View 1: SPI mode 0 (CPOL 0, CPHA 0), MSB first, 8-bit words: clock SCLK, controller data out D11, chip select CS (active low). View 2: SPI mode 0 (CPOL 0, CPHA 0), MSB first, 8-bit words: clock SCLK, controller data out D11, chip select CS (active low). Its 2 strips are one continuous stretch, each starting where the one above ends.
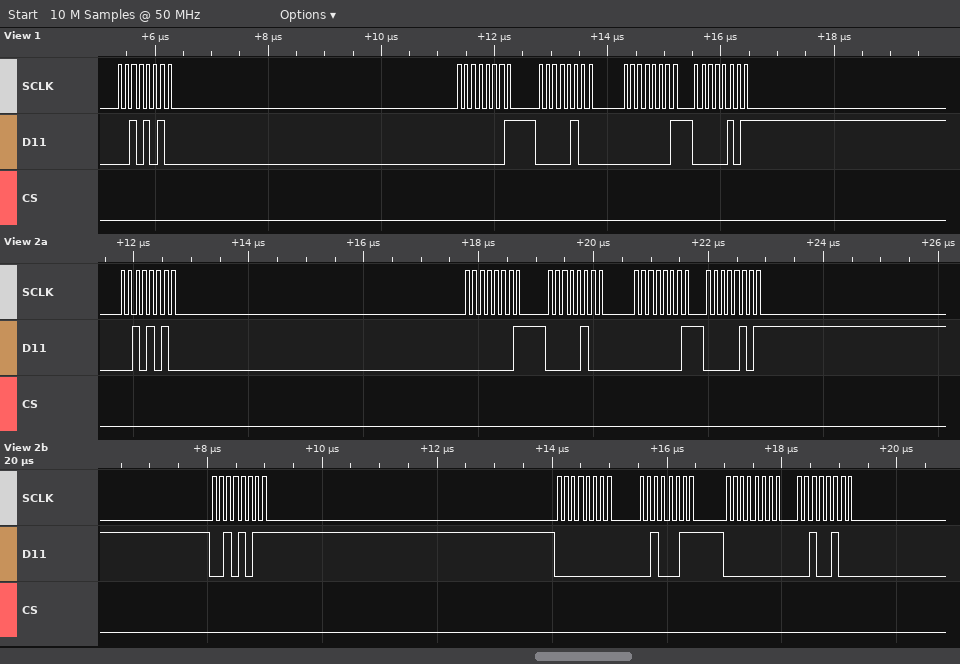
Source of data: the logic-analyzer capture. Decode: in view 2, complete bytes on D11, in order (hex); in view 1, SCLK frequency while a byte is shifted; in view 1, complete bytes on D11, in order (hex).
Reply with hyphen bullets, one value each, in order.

- 2A 01 04 01 05 2B 00 23 00 24
- 8 MHz
- 0x2A 0x01 0x04 0x01 0x05
